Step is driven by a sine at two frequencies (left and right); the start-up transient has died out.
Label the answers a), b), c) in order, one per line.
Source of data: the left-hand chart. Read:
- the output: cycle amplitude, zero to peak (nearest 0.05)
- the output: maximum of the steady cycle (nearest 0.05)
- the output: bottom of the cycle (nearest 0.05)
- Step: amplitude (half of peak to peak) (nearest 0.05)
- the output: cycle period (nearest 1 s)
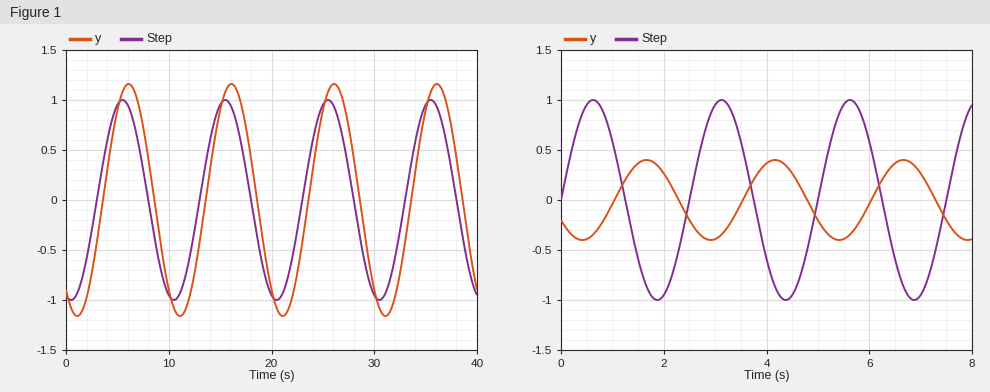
a) 1.15
b) 1.15
c) -1.15
d) 1.00
e) 10 s
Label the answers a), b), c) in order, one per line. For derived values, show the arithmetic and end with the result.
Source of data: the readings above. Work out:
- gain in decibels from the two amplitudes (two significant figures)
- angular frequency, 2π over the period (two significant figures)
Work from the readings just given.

a) 20 log10(1.15 / 1) = 1.2 dB
b) 2π / 10 = 0.63 rad/s
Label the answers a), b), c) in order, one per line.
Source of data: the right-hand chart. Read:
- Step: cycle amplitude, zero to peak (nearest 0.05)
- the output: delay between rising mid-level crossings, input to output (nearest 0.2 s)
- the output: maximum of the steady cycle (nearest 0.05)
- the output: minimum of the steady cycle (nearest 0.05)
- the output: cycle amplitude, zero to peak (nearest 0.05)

a) 1.00
b) 1.0 s
c) 0.40
d) -0.40
e) 0.40
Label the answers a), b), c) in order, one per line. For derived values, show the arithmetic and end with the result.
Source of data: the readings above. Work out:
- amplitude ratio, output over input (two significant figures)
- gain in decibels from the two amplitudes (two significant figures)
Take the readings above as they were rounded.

a) 0.4 / 1 = 0.40
b) 20 log10(0.4 / 1) = -8.0 dB
